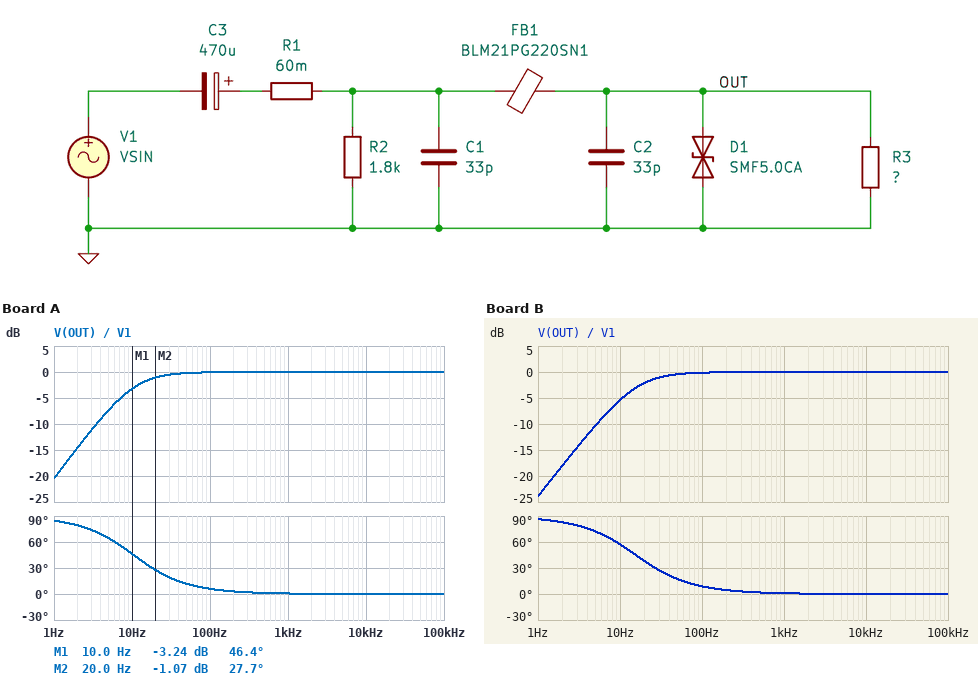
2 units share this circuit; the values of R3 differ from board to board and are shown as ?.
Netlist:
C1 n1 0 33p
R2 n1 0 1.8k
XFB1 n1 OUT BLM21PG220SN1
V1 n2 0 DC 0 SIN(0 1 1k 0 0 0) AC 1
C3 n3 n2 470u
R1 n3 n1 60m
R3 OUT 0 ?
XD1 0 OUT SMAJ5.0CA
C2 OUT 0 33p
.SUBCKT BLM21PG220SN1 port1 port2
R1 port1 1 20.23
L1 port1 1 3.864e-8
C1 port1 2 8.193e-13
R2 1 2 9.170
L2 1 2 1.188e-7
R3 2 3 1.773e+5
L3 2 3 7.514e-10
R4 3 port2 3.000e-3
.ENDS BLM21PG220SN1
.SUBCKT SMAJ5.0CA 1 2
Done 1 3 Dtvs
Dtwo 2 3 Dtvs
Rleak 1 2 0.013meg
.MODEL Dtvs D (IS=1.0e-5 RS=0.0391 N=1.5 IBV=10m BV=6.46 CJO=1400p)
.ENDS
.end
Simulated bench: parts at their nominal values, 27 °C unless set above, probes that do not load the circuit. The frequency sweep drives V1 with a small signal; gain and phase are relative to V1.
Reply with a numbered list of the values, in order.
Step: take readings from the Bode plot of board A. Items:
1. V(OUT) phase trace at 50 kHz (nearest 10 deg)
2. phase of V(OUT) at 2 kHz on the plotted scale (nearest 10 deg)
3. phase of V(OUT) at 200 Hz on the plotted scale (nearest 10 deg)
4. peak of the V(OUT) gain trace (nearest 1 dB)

1. 0 deg
2. 0 deg
3. 0 deg
4. 0 dB
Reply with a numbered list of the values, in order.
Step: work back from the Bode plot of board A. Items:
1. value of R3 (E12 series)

1. 33 Ω
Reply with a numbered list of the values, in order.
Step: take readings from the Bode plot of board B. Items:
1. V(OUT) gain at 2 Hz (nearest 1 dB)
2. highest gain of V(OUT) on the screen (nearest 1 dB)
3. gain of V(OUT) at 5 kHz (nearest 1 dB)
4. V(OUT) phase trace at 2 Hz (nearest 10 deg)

1. -18 dB
2. 0 dB
3. 0 dB
4. 80 deg
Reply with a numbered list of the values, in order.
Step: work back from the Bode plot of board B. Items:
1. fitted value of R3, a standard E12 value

1. 22 Ω
